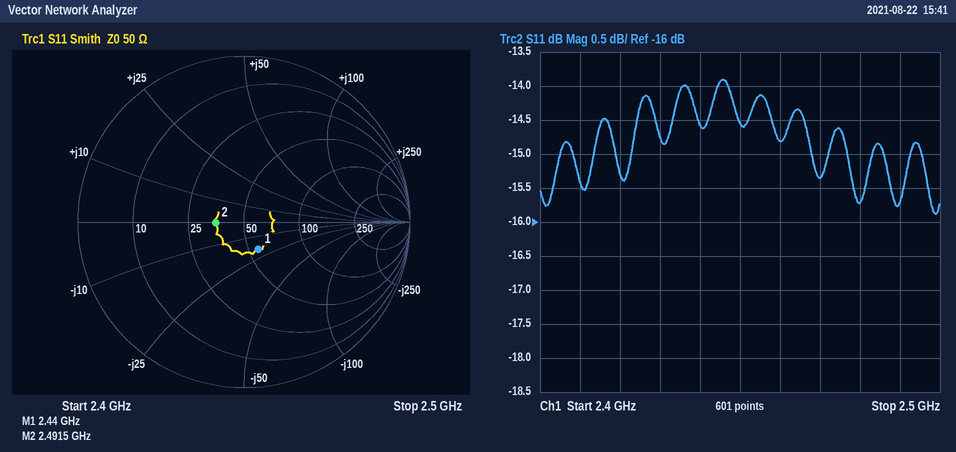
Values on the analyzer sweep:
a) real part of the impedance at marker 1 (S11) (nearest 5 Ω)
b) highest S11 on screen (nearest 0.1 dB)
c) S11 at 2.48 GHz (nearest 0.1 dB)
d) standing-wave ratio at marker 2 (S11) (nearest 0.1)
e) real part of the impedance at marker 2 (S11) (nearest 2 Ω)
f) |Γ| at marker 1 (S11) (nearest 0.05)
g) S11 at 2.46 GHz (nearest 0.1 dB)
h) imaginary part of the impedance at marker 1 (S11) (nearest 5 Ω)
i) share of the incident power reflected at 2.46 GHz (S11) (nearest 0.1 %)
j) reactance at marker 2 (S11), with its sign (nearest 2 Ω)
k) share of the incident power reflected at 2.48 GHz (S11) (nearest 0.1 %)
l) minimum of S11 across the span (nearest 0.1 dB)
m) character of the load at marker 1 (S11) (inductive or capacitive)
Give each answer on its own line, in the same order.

55 Ω
-13.9 dB
-15.7 dB
1.4
36 Ω
0.20
-14.8 dB
-20 Ω
3.3 %
0 Ω
2.7 %
-15.9 dB
capacitive
